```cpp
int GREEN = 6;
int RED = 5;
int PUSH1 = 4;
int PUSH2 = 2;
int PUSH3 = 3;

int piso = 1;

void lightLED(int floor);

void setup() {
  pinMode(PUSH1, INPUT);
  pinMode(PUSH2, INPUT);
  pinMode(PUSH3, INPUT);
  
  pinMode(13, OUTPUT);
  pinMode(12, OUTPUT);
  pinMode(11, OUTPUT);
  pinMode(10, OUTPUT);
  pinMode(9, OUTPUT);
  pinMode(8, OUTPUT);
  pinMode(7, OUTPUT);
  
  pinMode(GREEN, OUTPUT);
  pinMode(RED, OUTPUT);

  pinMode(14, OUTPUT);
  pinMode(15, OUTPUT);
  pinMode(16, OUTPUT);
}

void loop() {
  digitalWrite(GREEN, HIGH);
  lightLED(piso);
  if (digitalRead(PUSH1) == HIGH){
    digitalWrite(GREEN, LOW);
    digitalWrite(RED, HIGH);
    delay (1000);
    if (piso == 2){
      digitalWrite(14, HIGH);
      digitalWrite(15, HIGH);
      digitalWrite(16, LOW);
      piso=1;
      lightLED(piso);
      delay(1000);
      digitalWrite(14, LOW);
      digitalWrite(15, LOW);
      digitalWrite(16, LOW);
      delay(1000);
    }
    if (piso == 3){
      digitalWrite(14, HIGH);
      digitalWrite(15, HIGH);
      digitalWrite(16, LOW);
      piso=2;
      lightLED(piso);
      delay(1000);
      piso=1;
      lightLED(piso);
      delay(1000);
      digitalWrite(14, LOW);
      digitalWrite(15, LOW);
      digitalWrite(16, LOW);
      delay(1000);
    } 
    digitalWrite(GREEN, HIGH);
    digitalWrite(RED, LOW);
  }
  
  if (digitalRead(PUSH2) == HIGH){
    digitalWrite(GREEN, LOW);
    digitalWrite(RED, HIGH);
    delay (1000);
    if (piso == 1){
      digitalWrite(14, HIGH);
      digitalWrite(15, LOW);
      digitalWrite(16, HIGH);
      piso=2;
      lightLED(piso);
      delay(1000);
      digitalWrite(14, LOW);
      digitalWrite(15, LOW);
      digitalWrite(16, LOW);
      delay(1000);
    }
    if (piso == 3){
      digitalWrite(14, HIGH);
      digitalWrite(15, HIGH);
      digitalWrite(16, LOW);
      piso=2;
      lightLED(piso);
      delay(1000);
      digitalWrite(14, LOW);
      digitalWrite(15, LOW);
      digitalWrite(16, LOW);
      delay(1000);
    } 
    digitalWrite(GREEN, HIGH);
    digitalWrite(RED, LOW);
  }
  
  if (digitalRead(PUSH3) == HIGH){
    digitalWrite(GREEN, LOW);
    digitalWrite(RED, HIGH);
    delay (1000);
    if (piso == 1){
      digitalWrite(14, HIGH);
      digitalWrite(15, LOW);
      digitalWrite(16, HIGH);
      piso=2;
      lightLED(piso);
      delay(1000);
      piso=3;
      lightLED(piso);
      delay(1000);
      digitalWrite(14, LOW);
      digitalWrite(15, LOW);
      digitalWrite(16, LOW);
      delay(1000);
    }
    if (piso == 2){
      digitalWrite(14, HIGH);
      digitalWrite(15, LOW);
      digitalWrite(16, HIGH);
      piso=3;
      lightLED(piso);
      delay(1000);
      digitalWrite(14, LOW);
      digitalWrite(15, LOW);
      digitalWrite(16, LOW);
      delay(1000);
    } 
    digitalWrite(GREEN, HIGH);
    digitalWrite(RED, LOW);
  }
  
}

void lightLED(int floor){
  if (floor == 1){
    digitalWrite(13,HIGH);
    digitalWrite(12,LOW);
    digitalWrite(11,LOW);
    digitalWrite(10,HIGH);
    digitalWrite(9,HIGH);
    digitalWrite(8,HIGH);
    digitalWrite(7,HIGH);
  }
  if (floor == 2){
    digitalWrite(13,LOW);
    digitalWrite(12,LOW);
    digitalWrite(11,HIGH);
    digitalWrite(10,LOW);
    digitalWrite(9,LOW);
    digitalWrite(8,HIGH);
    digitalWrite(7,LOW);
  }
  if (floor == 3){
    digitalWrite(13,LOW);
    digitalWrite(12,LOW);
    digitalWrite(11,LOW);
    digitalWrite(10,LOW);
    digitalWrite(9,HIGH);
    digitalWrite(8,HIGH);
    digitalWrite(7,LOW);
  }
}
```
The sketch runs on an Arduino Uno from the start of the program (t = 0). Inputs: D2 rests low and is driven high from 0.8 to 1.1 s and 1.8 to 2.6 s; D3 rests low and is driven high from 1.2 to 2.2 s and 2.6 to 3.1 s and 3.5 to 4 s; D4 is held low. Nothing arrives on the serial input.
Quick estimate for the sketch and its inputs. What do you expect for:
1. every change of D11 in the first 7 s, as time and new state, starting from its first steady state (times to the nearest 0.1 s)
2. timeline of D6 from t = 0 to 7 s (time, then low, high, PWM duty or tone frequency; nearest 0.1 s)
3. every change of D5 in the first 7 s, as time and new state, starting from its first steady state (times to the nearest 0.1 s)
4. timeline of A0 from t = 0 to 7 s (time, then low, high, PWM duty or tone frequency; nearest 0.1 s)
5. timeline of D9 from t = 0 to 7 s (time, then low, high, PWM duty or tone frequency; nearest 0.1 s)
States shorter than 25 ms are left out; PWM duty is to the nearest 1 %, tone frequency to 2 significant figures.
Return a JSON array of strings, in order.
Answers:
["0 s low; 1.8 s high; 4.8 s low", "0 s high; 0.8 s low; 6.8 s high", "0 s low; 0.8 s high; 6.8 s low", "0 s low; 1.8 s high; 2.8 s low; 4.8 s high; 5.8 s low", "0 s high; 1.8 s low; 4.8 s high"]
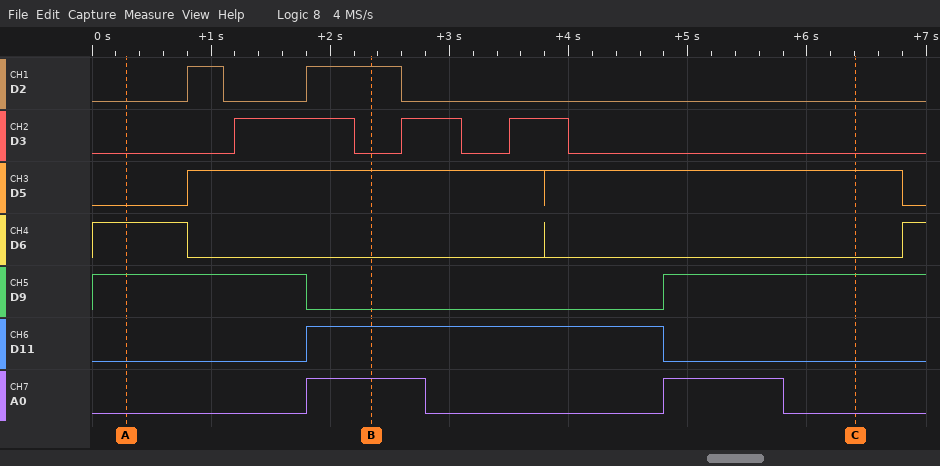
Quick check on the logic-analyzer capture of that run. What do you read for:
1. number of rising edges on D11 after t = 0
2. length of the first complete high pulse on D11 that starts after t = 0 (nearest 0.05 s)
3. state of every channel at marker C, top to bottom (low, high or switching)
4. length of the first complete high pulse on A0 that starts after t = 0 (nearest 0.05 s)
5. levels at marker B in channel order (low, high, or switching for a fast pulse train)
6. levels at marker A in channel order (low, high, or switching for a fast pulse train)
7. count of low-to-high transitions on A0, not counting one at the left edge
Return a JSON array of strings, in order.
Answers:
["1", "3.00 s", "D2 low, D3 low, D5 high, D6 low, D9 high, D11 low, A0 low", "1.00 s", "D2 high, D3 low, D5 high, D6 low, D9 low, D11 high, A0 high", "D2 low, D3 low, D5 low, D6 high, D9 high, D11 low, A0 low", "2"]
